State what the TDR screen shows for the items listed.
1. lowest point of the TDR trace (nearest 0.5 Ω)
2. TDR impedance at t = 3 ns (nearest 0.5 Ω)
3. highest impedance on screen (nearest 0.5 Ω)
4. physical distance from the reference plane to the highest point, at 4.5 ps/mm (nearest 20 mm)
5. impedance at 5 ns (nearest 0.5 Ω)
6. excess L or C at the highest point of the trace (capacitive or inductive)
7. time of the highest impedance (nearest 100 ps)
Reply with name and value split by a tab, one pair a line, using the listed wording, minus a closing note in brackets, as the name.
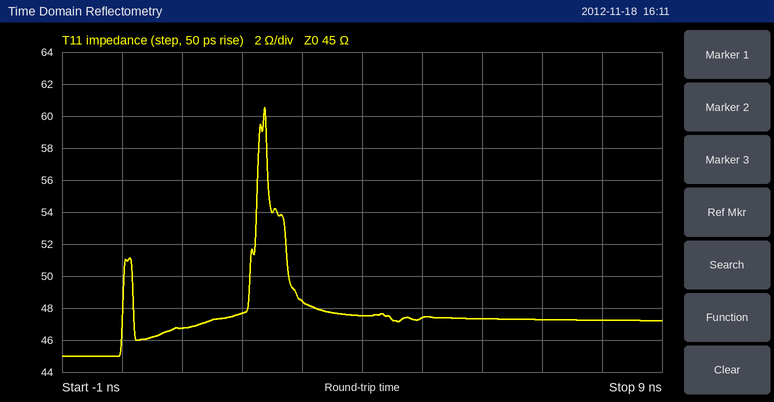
lowest point of the TDR trace	45.0 Ω
TDR impedance at t = 3 ns	48.5 Ω
highest impedance on screen	60.5 Ω
physical distance from the reference plane to the highest point, at 4.5 ps/mm	260 mm
impedance at 5 ns	47.5 Ω
excess L or C at the highest point of the trace	inductive
time of the highest impedance	2.4 ns
